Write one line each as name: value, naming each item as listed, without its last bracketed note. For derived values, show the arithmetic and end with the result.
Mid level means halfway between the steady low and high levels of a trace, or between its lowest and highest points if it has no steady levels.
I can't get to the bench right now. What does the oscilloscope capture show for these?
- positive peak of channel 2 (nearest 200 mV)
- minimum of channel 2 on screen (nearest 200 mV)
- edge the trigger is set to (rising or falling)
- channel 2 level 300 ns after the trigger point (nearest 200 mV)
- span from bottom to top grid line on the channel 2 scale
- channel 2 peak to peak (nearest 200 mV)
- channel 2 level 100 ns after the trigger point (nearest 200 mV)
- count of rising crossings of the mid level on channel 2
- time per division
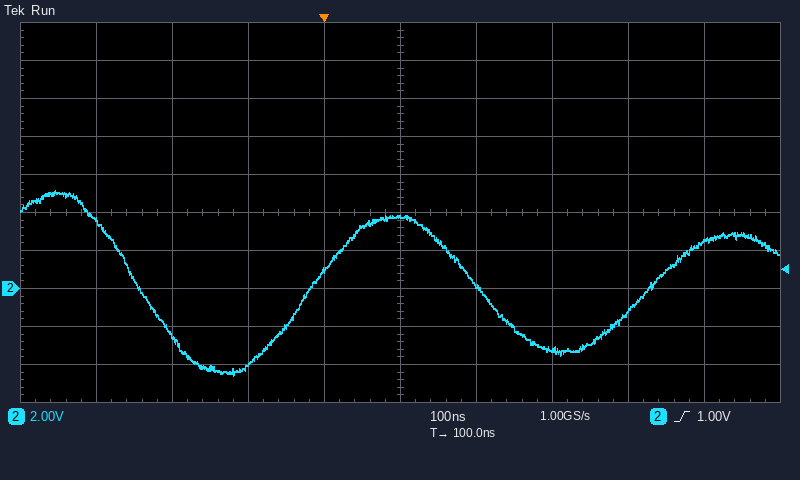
positive peak of channel 2: 5.2 V
minimum of channel 2 on screen: -4.6 V
edge the trigger is set to: rising
channel 2 level 300 ns after the trigger point: -3.2 V
span from bottom to top grid line on the channel 2 scale: 20 V
channel 2 peak to peak: 5.2 V − (-4.6 V) = 9.8 V
channel 2 level 100 ns after the trigger point: 3.8 V
count of rising crossings of the mid level on channel 2: 2
time per division: 100 ns
